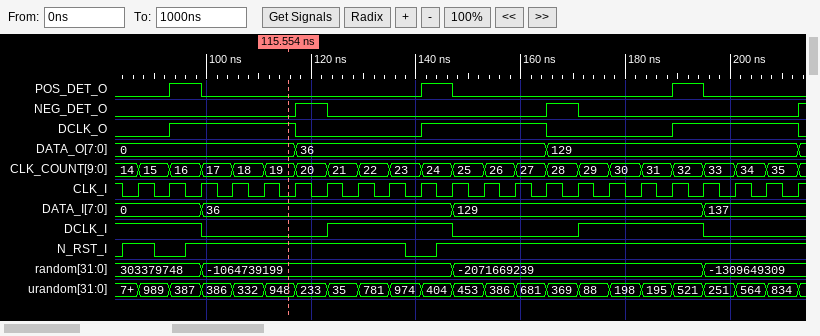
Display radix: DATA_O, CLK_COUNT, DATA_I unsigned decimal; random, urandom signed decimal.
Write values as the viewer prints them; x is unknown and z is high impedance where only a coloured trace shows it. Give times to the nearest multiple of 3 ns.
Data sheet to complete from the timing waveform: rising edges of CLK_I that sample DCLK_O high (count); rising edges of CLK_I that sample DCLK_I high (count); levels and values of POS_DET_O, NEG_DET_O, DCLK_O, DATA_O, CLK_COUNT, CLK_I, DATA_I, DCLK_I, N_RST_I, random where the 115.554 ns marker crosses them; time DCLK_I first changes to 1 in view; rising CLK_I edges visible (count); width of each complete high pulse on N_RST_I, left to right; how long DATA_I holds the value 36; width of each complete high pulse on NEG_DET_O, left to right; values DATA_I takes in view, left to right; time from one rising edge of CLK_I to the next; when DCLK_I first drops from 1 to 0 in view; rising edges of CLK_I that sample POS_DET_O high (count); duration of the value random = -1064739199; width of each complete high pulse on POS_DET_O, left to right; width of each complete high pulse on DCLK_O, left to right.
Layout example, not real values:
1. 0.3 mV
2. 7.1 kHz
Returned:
1. 12
2. 11
3. POS_DET_O=0, NEG_DET_O=0, DCLK_O=1, DATA_O=0, CLK_COUNT=19, CLK_I=0, DATA_I=36, DCLK_I=0, N_RST_I=1, random=-1064739199
4. 123 ns
5. 22
6. 6 ns, 42 ns
7. 48 ns
8. 6 ns, 6 ns
9. 0, 36, 129, 137
10. 6 ns
11. 99 ns
12. 3
13. 48 ns
14. 6 ns, 6 ns, 6 ns
15. 24 ns, 24 ns, 24 ns
